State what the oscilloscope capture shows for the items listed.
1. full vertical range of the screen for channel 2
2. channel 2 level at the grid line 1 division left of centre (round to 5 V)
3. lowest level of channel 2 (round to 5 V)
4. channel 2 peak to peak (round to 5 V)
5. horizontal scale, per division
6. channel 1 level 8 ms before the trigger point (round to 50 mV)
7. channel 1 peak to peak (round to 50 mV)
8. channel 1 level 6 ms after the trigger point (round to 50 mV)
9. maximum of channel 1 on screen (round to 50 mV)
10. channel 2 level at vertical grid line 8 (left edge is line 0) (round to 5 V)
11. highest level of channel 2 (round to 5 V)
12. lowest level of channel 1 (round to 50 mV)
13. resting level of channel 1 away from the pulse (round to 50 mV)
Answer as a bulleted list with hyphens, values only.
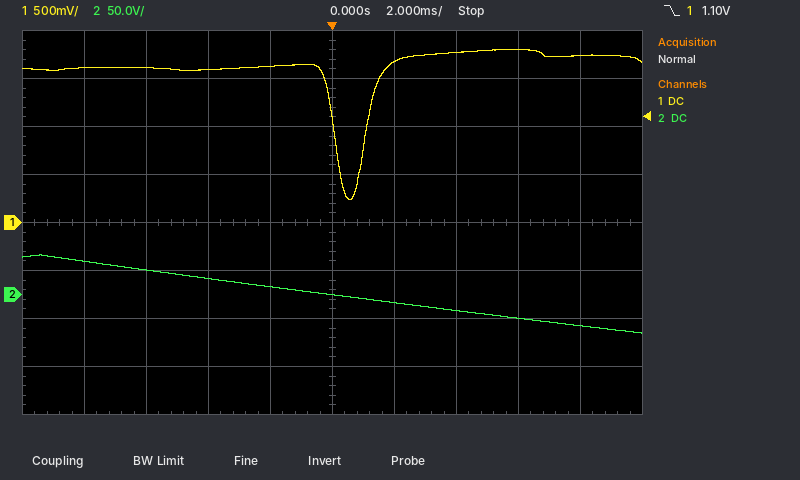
- 400 V
- 10 V
- -40 V
- 80 V
- 2 ms
- 1.60 V
- 1.55 V
- 1.80 V
- 1.80 V
- -25 V
- 40 V
- 250 mV
- 1.60 V
